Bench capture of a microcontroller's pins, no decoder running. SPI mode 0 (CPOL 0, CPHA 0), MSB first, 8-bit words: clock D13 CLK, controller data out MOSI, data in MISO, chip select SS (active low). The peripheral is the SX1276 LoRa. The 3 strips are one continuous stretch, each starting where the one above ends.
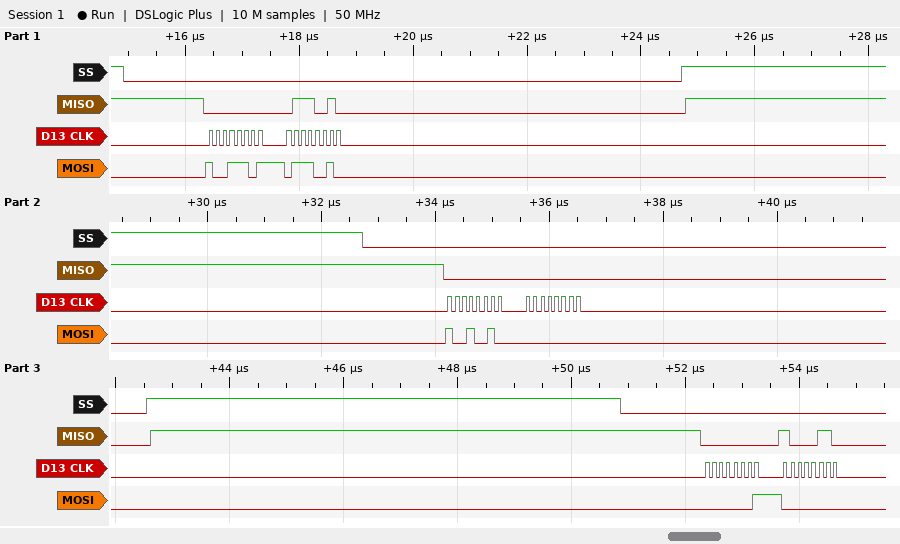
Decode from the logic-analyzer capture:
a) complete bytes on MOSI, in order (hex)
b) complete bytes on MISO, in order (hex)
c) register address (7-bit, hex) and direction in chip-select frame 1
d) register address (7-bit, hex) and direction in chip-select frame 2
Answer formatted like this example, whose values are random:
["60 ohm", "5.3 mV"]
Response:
["0x9D 0x72 0x92 0x00 0x01 0x00", "0x00 0x72 0x00 0x00 0x00 0x86", "0x1D write", "0x12 write"]
